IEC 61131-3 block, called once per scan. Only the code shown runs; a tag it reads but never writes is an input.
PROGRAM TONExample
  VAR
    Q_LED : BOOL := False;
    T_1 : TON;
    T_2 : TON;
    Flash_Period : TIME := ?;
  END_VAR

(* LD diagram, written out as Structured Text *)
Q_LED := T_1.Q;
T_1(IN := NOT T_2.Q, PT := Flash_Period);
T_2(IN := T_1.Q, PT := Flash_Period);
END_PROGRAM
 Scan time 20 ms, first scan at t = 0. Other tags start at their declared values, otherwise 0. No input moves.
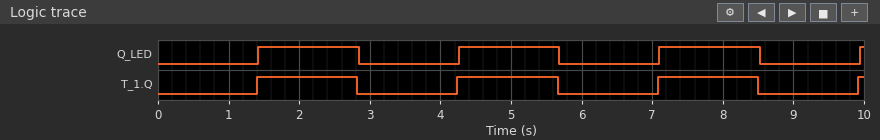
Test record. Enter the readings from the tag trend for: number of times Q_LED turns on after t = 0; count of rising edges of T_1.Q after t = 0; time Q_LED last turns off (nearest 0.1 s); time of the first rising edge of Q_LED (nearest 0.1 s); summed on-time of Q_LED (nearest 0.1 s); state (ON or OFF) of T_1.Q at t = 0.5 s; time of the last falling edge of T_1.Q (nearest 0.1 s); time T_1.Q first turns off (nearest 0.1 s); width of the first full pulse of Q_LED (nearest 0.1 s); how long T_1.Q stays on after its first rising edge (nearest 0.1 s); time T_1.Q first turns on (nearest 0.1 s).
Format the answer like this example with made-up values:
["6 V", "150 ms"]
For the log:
["4", "4", "8.5 s", "1.4 s", "4.3 s", "OFF", "8.5 s", "2.8 s", "1.4 s", "1.4 s", "1.4 s"]
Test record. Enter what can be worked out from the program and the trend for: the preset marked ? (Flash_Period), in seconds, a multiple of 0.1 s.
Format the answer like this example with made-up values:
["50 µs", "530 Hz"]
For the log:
["1.4 s"]
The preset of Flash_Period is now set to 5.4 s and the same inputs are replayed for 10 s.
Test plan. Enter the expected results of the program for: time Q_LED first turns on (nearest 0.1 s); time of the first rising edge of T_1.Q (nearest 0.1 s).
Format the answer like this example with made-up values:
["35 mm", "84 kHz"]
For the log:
["5.4 s", "5.4 s"]
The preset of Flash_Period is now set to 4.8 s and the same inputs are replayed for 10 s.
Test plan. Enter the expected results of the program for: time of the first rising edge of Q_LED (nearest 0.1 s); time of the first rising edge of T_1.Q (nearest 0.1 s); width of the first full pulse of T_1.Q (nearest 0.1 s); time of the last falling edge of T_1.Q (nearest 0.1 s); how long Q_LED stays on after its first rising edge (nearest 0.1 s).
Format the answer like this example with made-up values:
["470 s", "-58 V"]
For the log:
["4.8 s", "4.8 s", "4.8 s", "9.6 s", "4.8 s"]
